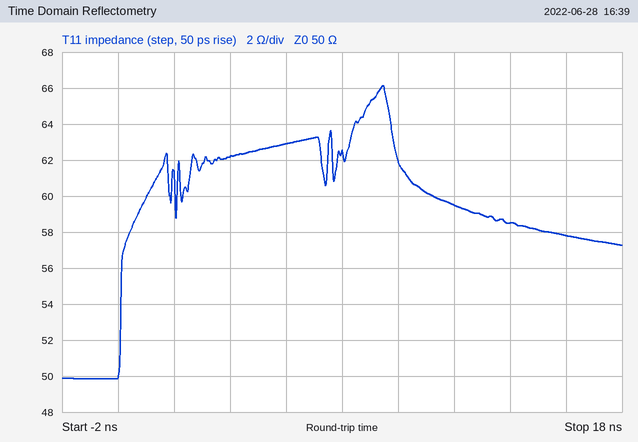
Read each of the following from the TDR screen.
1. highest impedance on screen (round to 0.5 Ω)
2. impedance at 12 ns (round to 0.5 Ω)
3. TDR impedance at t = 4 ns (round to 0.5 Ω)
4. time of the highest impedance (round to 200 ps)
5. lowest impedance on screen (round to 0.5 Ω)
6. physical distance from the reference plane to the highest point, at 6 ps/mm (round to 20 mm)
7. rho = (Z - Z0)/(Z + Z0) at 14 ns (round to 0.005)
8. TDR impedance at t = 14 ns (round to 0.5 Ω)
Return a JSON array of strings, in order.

["66.0 Ω", "59.5 Ω", "62.0 Ω", "9.4 ns", "50.0 Ω", "780 mm", "+0.080", "58.5 Ω"]
